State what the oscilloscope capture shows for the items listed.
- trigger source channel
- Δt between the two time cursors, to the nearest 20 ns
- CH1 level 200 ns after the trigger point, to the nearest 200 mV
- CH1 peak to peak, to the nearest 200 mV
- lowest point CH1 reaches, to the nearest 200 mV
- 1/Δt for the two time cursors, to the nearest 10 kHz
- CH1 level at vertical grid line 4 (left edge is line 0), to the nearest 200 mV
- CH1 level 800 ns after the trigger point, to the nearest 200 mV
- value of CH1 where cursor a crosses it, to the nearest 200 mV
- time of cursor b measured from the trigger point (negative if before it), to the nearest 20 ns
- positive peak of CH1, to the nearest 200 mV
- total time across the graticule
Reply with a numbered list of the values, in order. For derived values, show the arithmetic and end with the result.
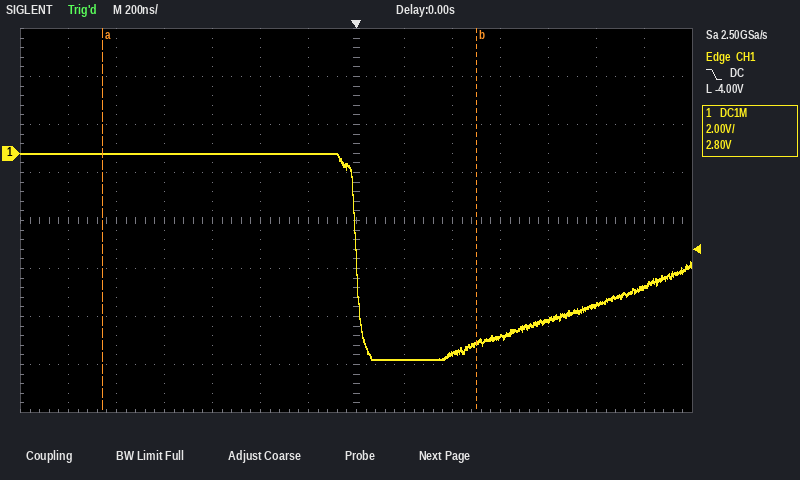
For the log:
1. CH1
2. 1.56 µs
3. -8.6 V
4. 0.0 V − (-8.6 V) = 8.6 V
5. -8.6 V
6. 1 / 1.56 µs ≈ 640 kHz
7. 0.0 V
8. -7.0 V
9. 0.0 V
10. +500 ns
11. 0.0 V
12. 2.8 µs
